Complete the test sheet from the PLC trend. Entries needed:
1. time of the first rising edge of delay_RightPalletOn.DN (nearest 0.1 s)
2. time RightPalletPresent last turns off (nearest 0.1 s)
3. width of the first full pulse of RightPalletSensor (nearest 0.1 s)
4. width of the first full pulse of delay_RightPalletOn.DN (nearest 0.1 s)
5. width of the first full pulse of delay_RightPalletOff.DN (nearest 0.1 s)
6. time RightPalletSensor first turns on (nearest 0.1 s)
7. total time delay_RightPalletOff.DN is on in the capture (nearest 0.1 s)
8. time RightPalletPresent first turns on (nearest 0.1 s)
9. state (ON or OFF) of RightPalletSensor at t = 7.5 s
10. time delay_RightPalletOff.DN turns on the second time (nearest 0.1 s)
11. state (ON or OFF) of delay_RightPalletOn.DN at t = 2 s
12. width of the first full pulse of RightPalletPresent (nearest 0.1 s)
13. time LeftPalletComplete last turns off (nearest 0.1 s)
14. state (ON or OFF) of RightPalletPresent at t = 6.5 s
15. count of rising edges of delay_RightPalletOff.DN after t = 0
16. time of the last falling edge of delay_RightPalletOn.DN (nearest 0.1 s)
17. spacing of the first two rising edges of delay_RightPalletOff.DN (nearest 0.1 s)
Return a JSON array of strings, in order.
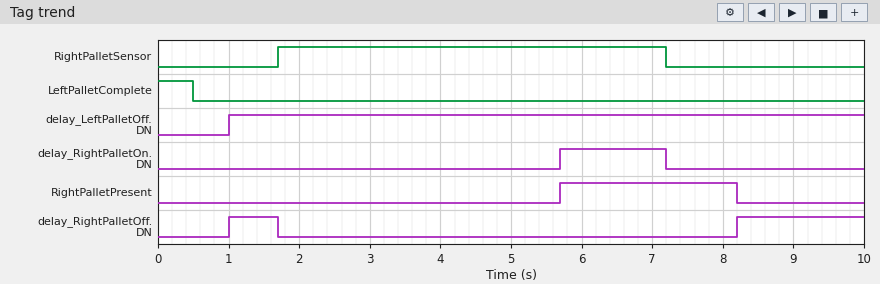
["5.7 s", "8.2 s", "5.5 s", "1.5 s", "0.7 s", "1.7 s", "2.5 s", "5.7 s", "OFF", "8.2 s", "OFF", "2.5 s", "0.5 s", "ON", "2", "7.2 s", "7.2 s"]
